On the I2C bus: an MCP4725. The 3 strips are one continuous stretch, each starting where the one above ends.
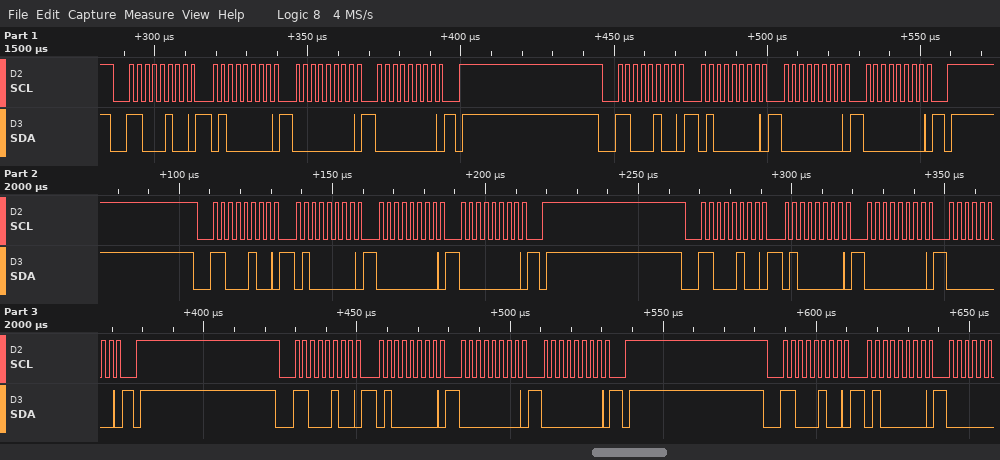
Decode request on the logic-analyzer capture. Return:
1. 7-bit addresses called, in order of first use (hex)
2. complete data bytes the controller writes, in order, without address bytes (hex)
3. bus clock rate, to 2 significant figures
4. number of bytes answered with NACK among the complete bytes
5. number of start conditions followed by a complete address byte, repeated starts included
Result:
0x62
40 00 00 40 00 00 40 00 00 40 00 00 40 00 00 40
400 kHz
0
6
